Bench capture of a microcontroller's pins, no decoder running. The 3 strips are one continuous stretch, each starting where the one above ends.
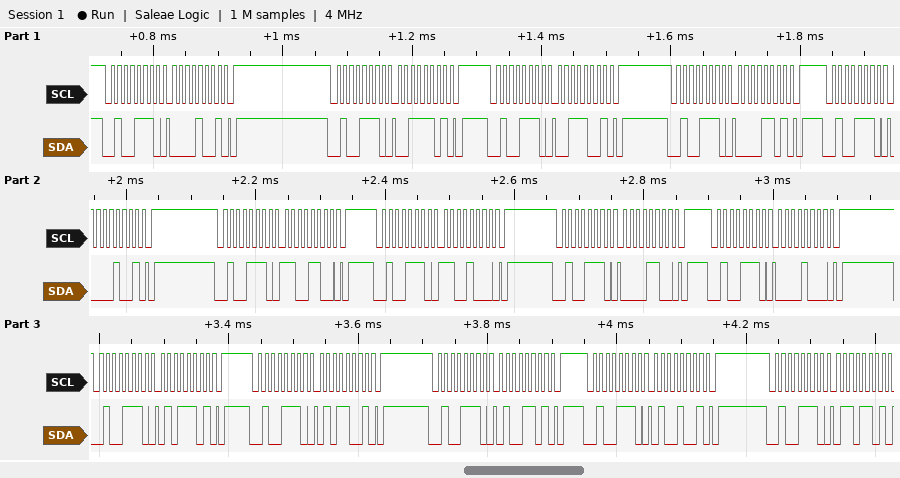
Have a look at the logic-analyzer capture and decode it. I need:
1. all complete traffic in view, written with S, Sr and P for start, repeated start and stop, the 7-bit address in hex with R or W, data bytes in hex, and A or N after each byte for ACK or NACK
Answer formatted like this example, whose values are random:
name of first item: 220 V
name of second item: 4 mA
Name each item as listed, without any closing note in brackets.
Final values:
all complete traffic in view, written with S, Sr and P for start, repeated start and stop, the 7-bit address in hex with R or W, data bytes in hex, and A or N after each byte for ACK or NACK: S 27W A 09 A P S 27W A 3D A P S 27W A 39 A P S 27W A 0D A P S 27W A 09 A P S 27W A CC A P S 27W A C8 A P S 27W A 0C A P S 27W A 08 A P S 27W A 5D A P S 27W A 59 A P S 27W A 4D A P S 27W A 49 A P S 27W A 6D A
